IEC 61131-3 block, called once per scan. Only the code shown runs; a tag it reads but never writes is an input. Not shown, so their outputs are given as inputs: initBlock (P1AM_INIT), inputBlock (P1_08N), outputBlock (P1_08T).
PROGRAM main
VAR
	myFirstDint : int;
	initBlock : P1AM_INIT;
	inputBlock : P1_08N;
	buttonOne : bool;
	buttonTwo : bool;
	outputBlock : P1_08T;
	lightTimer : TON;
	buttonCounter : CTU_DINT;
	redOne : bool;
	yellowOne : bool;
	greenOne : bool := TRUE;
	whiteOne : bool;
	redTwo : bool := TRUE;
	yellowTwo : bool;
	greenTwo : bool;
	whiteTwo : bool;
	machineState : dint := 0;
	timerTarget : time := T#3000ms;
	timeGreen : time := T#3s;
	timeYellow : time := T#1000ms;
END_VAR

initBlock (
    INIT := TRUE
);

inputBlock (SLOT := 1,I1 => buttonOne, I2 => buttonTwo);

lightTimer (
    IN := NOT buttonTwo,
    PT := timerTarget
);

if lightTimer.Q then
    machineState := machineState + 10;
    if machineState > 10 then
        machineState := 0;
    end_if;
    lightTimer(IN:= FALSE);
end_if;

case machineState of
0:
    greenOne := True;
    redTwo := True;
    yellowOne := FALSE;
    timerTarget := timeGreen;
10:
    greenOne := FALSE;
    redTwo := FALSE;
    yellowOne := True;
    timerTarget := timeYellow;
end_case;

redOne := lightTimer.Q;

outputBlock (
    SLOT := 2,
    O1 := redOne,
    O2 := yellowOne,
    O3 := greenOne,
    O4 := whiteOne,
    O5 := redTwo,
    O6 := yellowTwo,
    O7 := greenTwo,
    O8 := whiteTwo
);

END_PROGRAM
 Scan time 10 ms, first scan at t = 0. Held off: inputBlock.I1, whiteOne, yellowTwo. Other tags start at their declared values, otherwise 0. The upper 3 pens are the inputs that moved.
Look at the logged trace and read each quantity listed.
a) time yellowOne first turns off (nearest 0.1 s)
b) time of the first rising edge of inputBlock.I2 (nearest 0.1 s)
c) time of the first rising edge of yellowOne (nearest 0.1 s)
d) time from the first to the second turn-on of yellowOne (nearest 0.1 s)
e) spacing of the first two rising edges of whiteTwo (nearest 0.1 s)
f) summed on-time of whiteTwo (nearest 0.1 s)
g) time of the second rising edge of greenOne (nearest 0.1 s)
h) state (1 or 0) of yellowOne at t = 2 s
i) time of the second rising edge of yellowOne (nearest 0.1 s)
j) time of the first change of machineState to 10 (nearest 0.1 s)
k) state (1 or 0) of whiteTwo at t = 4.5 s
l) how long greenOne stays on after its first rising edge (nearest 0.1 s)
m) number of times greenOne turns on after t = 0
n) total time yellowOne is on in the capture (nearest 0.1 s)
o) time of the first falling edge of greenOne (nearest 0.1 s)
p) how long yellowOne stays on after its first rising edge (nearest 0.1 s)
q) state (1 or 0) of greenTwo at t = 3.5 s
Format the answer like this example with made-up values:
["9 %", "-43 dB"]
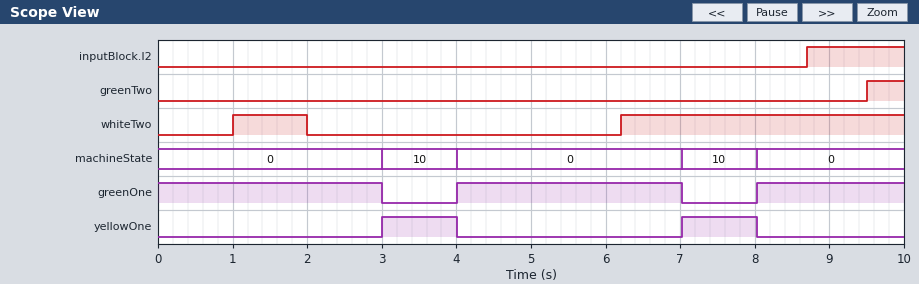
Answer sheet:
["4.0 s", "8.7 s", "3.0 s", "4.0 s", "5.2 s", "4.8 s", "8.0 s", "0", "7.0 s", "3.0 s", "0", "3.0 s", "2", "2.0 s", "3.0 s", "1.0 s", "0"]
